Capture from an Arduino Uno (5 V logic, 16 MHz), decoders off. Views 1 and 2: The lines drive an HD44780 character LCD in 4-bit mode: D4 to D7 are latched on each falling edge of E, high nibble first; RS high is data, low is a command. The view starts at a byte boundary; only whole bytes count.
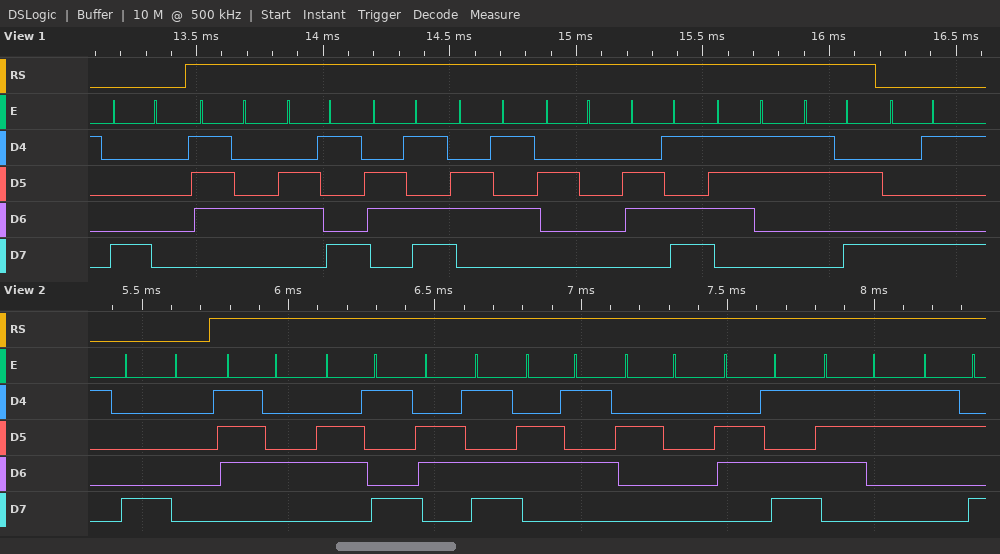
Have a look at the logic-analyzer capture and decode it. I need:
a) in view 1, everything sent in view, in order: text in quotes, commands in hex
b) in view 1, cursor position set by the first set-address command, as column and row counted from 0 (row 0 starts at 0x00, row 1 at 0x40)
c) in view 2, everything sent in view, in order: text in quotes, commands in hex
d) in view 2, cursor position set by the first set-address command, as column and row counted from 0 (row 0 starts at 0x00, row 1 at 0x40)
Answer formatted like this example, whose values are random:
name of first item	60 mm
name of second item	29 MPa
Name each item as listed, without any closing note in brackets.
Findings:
in view 1, everything sent in view, in order: text in quotes, commands in hex	0x80 "time ms:" 0x89
in view 1, cursor position set by the first set-address command, as column and row counted from 0	column 0, row 0
in view 2, everything sent in view, in order: text in quotes, commands in hex	0x80 "time ms:"
in view 2, cursor position set by the first set-address command, as column and row counted from 0	column 0, row 0
